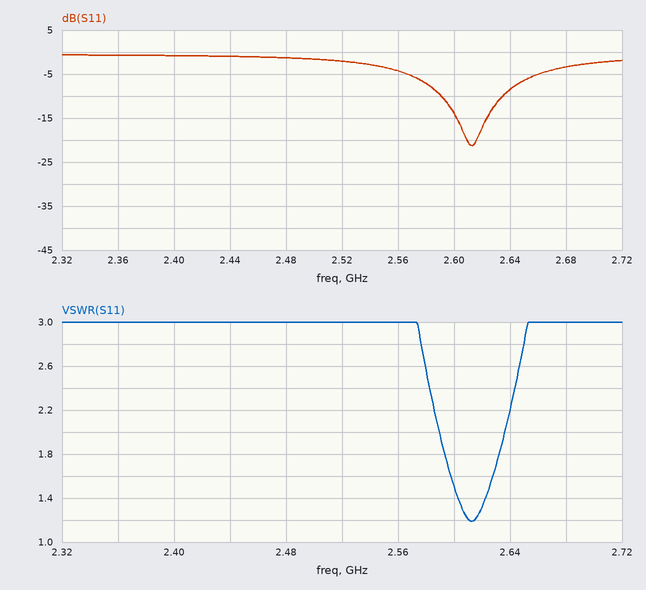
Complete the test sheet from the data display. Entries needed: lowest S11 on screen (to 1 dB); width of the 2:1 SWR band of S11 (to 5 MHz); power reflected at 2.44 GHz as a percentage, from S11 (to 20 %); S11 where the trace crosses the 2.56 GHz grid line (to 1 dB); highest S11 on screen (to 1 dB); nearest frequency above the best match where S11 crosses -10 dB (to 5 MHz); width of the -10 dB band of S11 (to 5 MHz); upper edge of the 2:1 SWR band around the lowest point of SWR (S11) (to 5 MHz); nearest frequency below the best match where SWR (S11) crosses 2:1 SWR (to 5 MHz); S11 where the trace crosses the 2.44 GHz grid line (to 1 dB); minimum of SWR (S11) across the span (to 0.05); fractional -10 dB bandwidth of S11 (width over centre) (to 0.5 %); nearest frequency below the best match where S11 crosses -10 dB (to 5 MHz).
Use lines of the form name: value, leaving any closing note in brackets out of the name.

lowest S11 on screen: -21 dB
width of the 2:1 SWR band of S11: 45 MHz
power reflected at 2.44 GHz as a percentage, from S11: 80 %
S11 where the trace crosses the 2.56 GHz grid line: -4 dB
highest S11 on screen: -1 dB
nearest frequency above the best match where S11 crosses -10 dB: 2.635 GHz
width of the -10 dB band of S11: 45 MHz
upper edge of the 2:1 SWR band around the lowest point of SWR (S11): 2.635 GHz
nearest frequency below the best match where SWR (S11) crosses 2:1 SWR: 2.590 GHz
S11 where the trace crosses the 2.44 GHz grid line: -1 dB
minimum of SWR (S11) across the span: 1.20
fractional -10 dB bandwidth of S11 (width over centre): 1.5 %
nearest frequency below the best match where S11 crosses -10 dB: 2.590 GHz
